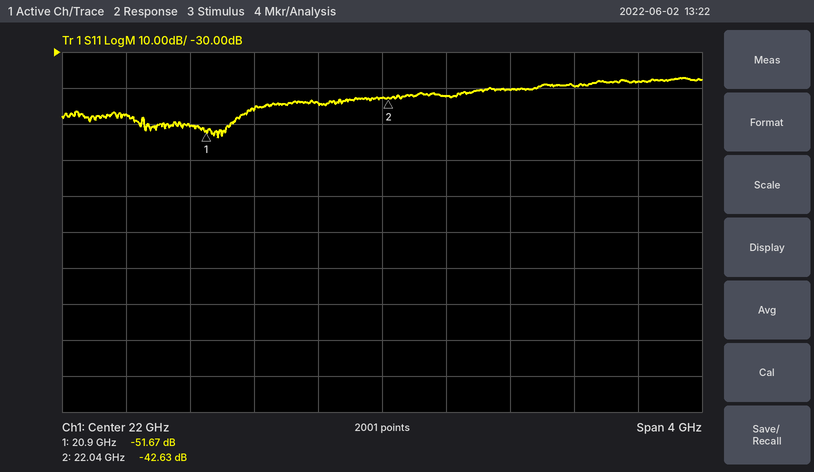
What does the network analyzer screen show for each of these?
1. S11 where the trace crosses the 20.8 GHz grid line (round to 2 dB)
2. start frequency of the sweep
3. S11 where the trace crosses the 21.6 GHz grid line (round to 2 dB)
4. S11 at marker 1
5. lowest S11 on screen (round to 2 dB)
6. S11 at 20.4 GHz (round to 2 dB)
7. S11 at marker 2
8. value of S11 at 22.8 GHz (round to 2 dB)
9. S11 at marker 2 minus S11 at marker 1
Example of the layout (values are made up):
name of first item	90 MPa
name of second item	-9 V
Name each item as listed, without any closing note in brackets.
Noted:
S11 where the trace crosses the 20.8 GHz grid line	-50 dB
start frequency of the sweep	20 GHz
S11 where the trace crosses the 21.6 GHz grid line	-44 dB
S11 at marker 1	-51.67 dB
lowest S11 on screen	-54 dB
S11 at 20.4 GHz	-48 dB
S11 at marker 2	-42.63 dB
value of S11 at 22.8 GHz	-40 dB
S11 at marker 2 minus S11 at marker 1	9.04 dB
